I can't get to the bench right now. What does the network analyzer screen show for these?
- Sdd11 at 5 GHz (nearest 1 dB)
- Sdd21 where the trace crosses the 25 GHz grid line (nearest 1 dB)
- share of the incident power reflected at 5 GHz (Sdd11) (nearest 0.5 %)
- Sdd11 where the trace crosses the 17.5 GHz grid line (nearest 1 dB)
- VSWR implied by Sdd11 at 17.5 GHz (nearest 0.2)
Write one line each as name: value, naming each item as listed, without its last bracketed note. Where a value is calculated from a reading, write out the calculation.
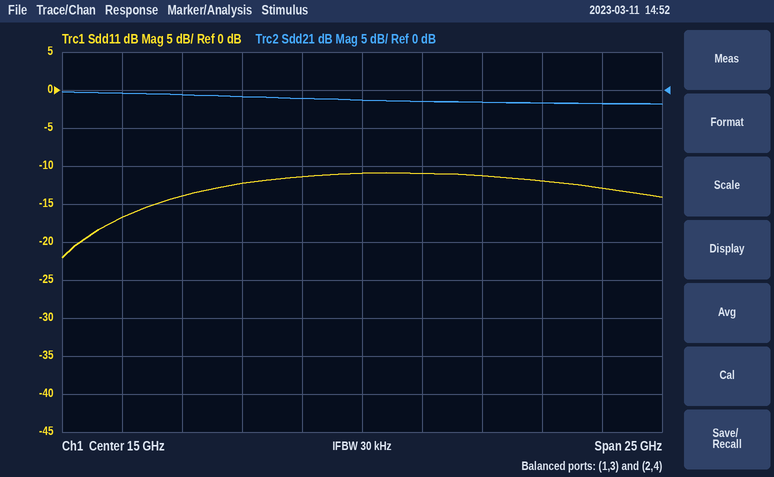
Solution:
Sdd11 at 5 GHz: -17 dB
Sdd21 where the trace crosses the 25 GHz grid line: -2 dB
share of the incident power reflected at 5 GHz (Sdd11): 10^(-17/10) ≈ 2.0 %
Sdd11 where the trace crosses the 17.5 GHz grid line: -11 dB
VSWR implied by Sdd11 at 17.5 GHz: |Γ| = 10^(-11/20) = 0.2818; VSWR = (1 + 0.2818)/(1 − 0.2818) ≈ 1.8
